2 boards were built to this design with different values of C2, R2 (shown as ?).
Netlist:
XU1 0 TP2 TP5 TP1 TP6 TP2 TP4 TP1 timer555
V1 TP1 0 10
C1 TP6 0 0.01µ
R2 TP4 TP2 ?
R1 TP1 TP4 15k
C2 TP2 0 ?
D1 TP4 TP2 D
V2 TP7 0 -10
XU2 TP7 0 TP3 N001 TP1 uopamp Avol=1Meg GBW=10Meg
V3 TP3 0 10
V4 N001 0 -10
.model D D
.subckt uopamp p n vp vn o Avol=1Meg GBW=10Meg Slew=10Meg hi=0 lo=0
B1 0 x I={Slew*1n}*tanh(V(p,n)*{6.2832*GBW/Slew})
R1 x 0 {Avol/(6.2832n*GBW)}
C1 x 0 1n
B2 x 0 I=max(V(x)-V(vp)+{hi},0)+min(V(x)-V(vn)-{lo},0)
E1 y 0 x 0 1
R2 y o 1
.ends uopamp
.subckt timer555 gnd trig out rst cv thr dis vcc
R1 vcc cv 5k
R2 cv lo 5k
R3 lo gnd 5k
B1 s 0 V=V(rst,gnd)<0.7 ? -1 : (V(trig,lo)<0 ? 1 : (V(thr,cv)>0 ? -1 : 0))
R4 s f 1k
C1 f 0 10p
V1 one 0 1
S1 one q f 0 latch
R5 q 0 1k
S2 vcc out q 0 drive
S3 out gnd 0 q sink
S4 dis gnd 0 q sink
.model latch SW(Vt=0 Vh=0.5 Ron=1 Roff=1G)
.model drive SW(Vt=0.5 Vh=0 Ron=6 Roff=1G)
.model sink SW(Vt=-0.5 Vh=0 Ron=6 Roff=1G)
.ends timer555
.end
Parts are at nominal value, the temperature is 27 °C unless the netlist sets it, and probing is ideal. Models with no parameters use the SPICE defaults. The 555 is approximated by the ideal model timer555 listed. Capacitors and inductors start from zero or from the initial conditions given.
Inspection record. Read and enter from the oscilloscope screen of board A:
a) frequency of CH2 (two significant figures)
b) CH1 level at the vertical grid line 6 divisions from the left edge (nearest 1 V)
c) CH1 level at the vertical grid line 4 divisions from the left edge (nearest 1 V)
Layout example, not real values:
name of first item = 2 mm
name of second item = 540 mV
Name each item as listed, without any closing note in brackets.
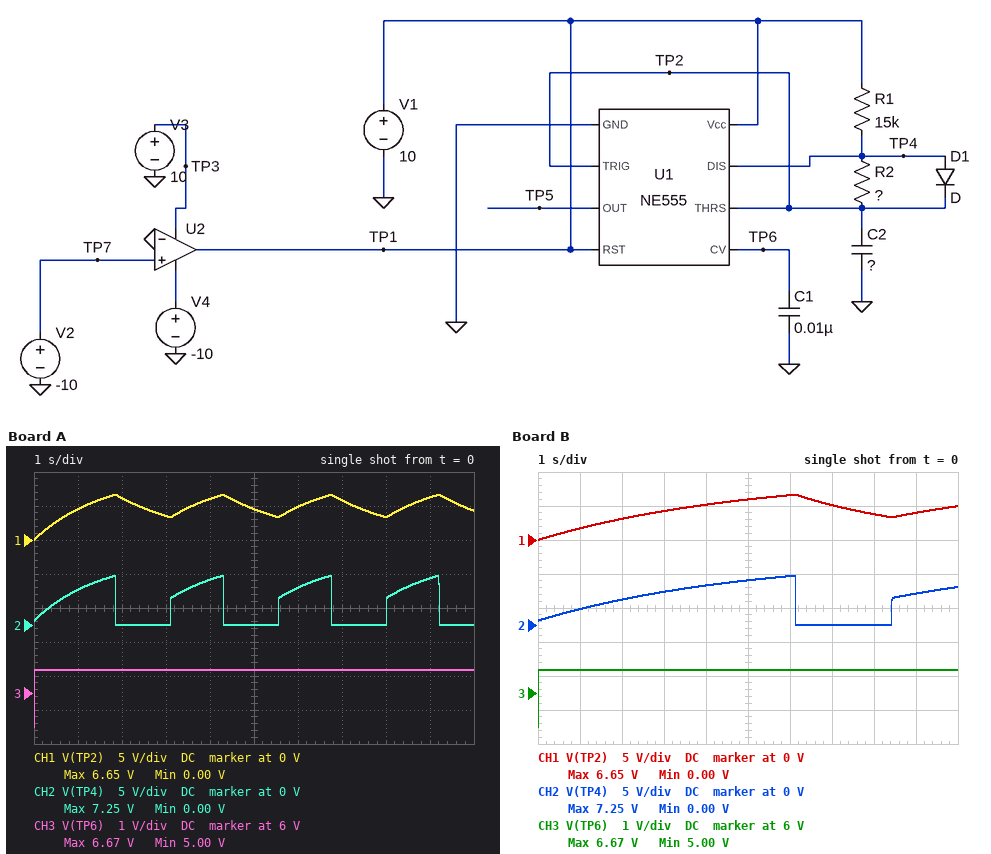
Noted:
frequency of CH2 = 400 mHz
CH1 level at the vertical grid line 6 divisions from the left edge = 5 V
CH1 level at the vertical grid line 4 divisions from the left edge = 6 V
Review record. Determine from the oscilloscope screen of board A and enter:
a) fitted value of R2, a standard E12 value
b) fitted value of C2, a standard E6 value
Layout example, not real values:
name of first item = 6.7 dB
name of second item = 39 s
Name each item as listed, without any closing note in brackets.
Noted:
fitted value of R2, a standard E12 value = 18 kΩ
fitted value of C2, a standard E6 value = 100 µF
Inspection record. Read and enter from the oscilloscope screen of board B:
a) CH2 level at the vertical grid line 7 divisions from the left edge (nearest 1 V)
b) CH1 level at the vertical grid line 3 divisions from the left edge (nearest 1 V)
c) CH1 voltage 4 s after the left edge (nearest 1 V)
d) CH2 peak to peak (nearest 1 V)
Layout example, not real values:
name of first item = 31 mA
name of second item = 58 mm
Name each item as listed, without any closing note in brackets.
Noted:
CH2 level at the vertical grid line 7 divisions from the left edge = 0 V
CH1 level at the vertical grid line 3 divisions from the left edge = 4 V
CH1 voltage 4 s after the left edge = 5 V
CH2 peak to peak = 7 V
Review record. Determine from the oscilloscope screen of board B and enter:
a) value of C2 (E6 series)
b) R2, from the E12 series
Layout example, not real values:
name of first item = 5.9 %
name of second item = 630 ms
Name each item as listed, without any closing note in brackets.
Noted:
value of C2 = 330 µF
R2, from the E12 series = 10 kΩ
